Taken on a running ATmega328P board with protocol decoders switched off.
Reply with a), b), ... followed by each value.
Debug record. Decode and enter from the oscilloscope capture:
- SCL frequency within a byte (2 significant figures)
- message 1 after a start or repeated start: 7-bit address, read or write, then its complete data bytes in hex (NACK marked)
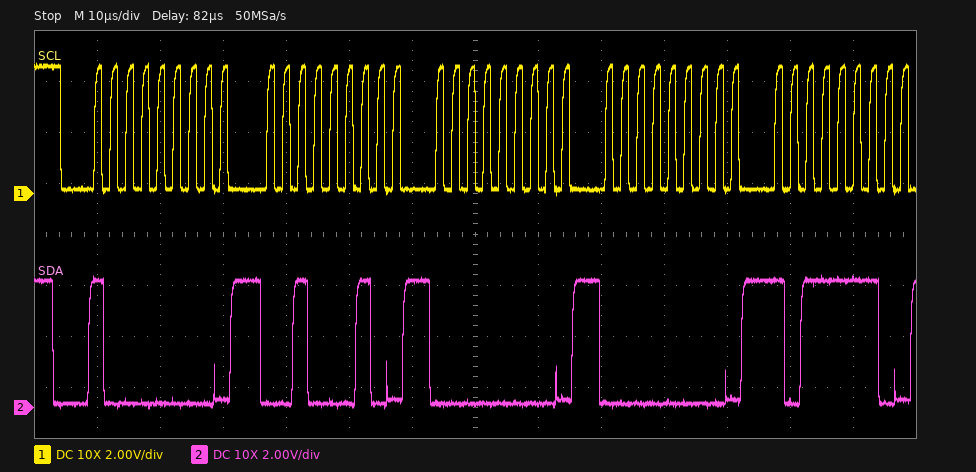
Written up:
a) 400 kHz
b) 0x40 write: 22 00 00 BE
